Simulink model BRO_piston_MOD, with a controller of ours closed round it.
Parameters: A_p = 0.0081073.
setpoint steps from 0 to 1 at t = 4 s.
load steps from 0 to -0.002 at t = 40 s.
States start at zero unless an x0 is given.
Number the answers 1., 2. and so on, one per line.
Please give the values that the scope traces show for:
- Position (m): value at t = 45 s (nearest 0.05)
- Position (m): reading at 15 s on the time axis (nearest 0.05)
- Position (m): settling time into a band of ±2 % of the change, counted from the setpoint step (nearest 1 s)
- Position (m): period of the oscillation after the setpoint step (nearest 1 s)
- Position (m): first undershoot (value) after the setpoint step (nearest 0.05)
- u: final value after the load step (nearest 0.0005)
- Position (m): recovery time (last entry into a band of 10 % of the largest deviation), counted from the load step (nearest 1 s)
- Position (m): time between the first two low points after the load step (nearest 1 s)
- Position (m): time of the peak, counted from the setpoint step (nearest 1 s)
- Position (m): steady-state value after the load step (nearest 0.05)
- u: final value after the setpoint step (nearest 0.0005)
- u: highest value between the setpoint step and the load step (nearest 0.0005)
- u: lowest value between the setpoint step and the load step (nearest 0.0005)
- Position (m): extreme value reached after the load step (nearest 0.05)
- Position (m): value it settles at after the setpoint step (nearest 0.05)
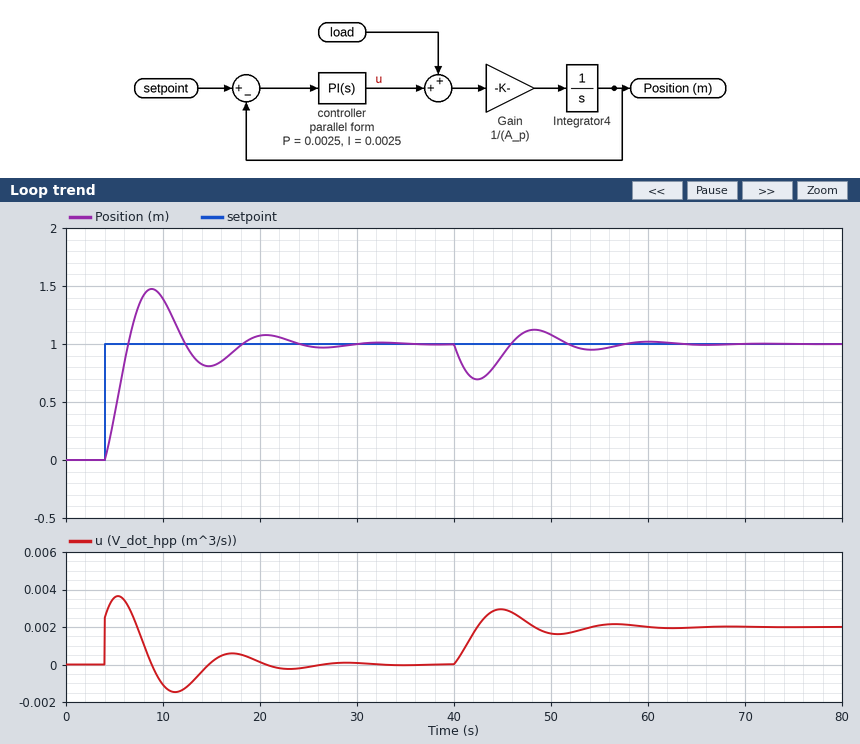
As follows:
1. 0.90
2. 0.80
3. 24 s
4. 12 s
5. 0.80
6. 0.0020
7. 16 s
8. 12 s
9. 5 s
10. 1.00
11. 0.0000
12. 0.0035
13. -0.0015
14. 0.70
15. 1.00
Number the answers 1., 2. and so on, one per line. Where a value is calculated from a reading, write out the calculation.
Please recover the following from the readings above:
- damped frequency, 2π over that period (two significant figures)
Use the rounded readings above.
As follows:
1. 2π / 12 = 0.52 rad/s
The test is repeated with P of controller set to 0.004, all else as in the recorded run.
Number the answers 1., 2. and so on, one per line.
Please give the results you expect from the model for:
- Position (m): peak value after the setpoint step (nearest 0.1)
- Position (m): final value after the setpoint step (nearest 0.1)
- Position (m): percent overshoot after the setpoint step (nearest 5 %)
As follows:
1. 1.3
2. 1.0
3. 35 %
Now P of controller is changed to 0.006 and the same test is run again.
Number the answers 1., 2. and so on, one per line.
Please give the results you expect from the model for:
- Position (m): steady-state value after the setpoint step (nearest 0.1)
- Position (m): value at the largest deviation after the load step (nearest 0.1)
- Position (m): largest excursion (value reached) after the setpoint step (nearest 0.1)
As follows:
1. 1.0
2. 0.8
3. 1.2
